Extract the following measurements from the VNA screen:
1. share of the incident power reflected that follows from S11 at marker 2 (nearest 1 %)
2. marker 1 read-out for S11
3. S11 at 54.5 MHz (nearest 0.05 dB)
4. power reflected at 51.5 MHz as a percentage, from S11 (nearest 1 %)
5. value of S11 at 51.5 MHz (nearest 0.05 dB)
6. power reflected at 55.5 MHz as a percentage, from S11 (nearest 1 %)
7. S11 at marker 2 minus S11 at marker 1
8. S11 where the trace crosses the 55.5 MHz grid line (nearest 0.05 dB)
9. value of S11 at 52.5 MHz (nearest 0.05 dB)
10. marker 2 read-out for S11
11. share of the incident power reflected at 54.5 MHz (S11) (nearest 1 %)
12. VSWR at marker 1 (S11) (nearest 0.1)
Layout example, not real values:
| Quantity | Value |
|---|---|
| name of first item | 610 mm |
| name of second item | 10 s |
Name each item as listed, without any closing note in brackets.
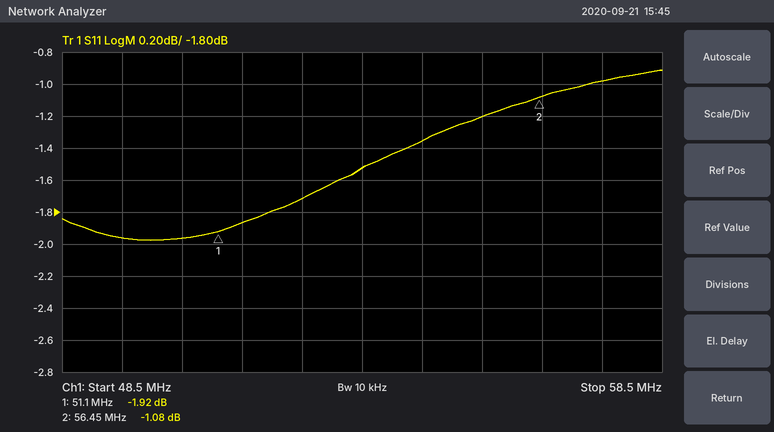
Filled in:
| Quantity | Value |
|---|---|
| share of the incident power reflected that follows from S11 at marker 2 | 78 % |
| marker 1 read-out for S11 | -1.92 dB |
| S11 at 54.5 MHz | -1.35 dB |
| power reflected at 51.5 MHz as a percentage, from S11 | 65 % |
| value of S11 at 51.5 MHz | -1.85 dB |
| power reflected at 55.5 MHz as a percentage, from S11 | 76 % |
| S11 at marker 2 minus S11 at marker 1 | 0.84 dB |
| S11 where the trace crosses the 55.5 MHz grid line | -1.20 dB |
| value of S11 at 52.5 MHz | -1.70 dB |
| marker 2 read-out for S11 | -1.08 dB |
| share of the incident power reflected at 54.5 MHz (S11) | 73 % |
| VSWR at marker 1 (S11) | 9.1 |
